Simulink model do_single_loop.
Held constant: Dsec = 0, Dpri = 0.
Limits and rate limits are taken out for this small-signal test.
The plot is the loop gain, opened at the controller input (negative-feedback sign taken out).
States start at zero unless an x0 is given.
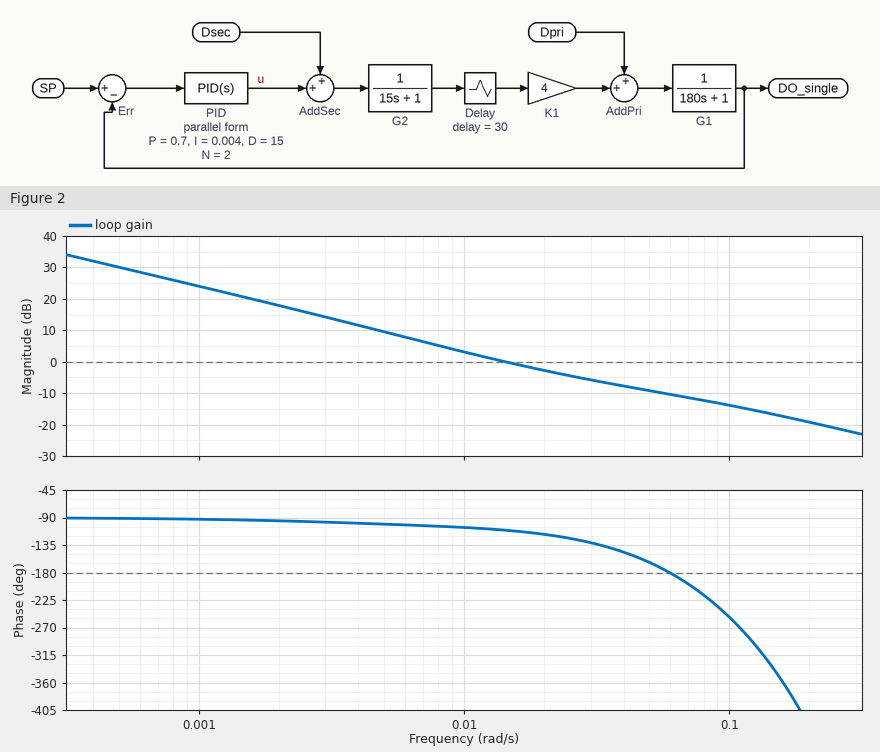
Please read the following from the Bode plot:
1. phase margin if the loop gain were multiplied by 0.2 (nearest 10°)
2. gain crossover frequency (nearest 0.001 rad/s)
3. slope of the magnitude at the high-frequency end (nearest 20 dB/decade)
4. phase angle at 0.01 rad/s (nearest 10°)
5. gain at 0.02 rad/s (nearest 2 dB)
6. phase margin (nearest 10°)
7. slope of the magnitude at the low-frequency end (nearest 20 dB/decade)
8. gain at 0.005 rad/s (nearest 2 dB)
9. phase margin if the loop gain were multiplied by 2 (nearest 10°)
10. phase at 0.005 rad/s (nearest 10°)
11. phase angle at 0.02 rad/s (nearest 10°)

80°
0.014 rad/s
-20 dB/decade
-110°
-2 dB
70°
-20 dB/decade
10 dB
50°
-100°
-120°
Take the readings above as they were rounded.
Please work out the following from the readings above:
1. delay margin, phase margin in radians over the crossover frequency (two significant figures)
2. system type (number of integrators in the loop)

87 s
1
